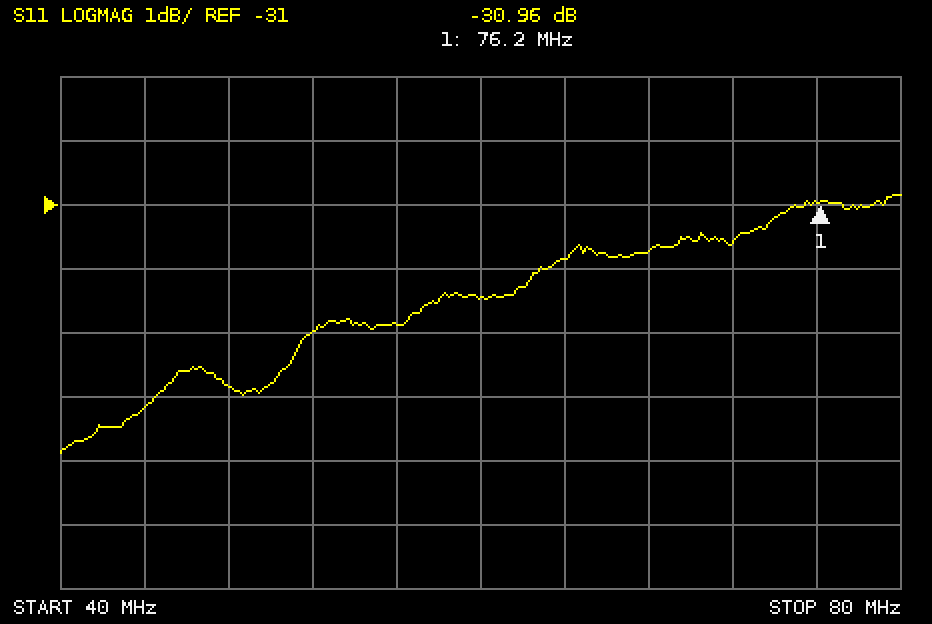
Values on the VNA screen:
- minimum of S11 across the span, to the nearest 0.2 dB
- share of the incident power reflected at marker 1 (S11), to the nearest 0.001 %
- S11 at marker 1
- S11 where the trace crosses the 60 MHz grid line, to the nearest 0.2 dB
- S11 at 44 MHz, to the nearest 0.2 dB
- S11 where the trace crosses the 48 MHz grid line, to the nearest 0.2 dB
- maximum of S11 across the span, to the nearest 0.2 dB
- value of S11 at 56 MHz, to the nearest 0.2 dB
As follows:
-34.8 dB
0.080 %
-30.96 dB
-32.4 dB
-34.2 dB
-33.8 dB
-30.8 dB
-32.8 dB
